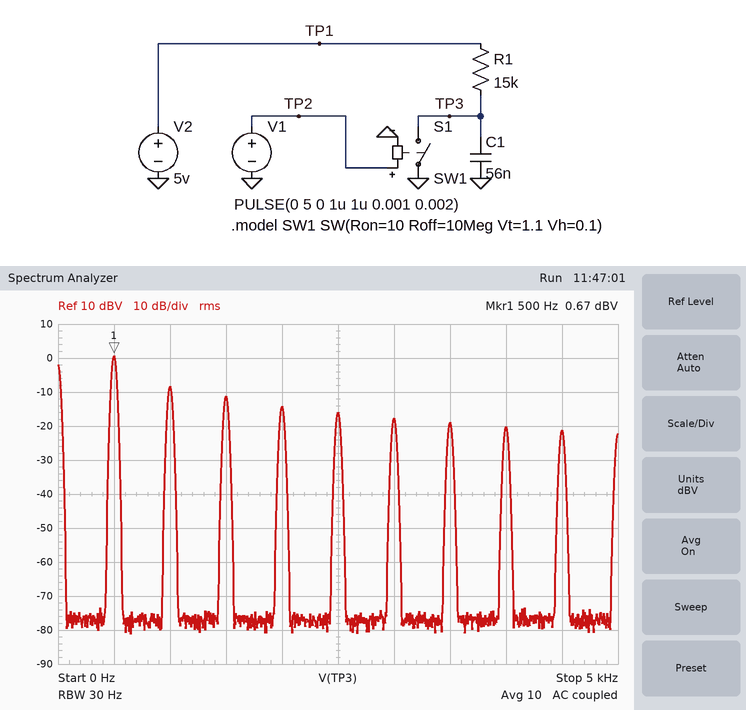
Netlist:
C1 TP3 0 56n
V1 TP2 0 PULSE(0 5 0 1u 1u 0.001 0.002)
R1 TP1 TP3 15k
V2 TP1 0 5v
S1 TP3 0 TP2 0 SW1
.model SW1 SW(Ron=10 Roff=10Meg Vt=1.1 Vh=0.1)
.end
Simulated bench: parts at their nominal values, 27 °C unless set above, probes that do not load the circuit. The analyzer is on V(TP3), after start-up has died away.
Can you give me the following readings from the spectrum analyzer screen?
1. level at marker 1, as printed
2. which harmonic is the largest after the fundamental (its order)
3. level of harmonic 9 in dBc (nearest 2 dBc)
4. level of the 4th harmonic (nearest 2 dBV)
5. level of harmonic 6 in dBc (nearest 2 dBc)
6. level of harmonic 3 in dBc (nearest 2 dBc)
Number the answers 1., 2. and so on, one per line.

1. 0.67 dBV
2. 2
3. -22 dBc
4. -14 dBV
5. -18 dBc
6. -12 dBc
